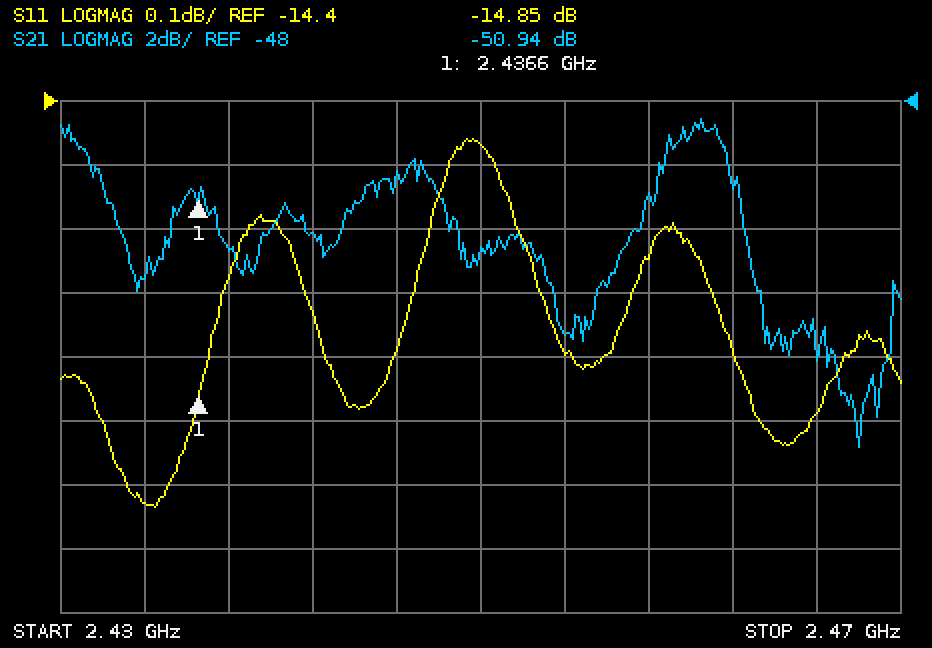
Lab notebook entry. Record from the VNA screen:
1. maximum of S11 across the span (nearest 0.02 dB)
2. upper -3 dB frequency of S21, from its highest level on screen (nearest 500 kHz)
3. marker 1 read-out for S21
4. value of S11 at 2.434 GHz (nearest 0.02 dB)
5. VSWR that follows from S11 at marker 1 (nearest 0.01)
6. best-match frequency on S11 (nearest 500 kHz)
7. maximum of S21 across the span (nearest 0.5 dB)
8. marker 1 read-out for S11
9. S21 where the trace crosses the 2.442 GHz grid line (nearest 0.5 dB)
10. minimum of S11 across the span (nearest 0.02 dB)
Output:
-14.46 dB
2.4625 GHz
-50.94 dB
-15.02 dB
1.44
2.4345 GHz
-48.5 dB
-14.85 dB
-52.0 dB
-15.04 dB
